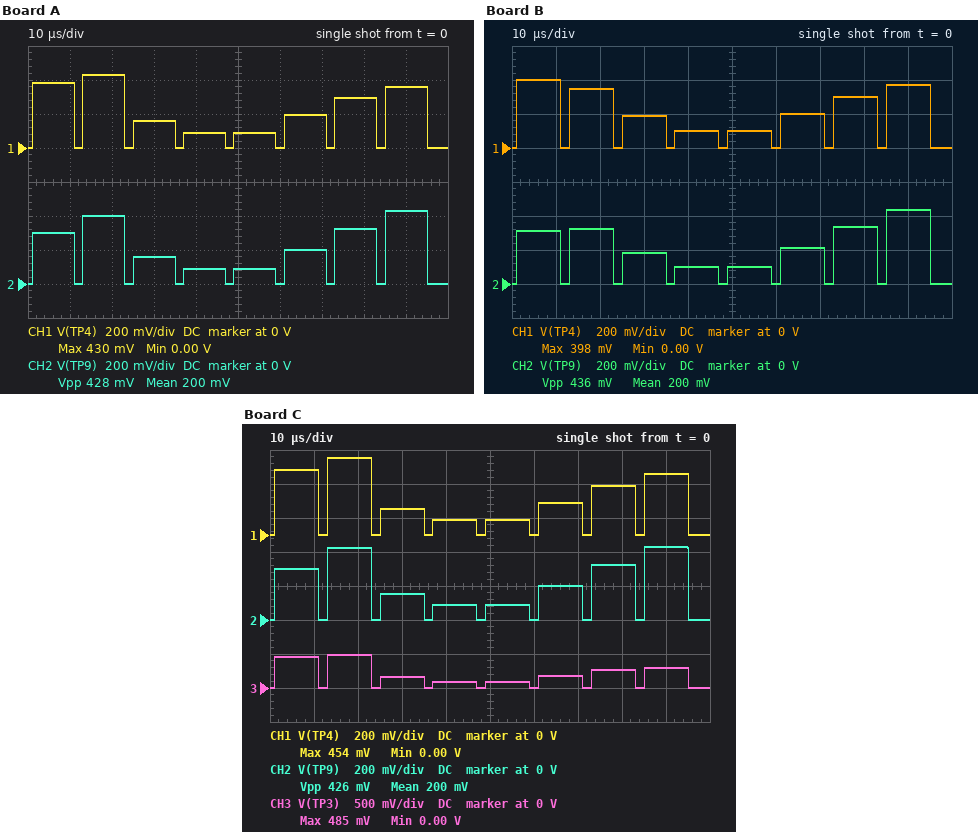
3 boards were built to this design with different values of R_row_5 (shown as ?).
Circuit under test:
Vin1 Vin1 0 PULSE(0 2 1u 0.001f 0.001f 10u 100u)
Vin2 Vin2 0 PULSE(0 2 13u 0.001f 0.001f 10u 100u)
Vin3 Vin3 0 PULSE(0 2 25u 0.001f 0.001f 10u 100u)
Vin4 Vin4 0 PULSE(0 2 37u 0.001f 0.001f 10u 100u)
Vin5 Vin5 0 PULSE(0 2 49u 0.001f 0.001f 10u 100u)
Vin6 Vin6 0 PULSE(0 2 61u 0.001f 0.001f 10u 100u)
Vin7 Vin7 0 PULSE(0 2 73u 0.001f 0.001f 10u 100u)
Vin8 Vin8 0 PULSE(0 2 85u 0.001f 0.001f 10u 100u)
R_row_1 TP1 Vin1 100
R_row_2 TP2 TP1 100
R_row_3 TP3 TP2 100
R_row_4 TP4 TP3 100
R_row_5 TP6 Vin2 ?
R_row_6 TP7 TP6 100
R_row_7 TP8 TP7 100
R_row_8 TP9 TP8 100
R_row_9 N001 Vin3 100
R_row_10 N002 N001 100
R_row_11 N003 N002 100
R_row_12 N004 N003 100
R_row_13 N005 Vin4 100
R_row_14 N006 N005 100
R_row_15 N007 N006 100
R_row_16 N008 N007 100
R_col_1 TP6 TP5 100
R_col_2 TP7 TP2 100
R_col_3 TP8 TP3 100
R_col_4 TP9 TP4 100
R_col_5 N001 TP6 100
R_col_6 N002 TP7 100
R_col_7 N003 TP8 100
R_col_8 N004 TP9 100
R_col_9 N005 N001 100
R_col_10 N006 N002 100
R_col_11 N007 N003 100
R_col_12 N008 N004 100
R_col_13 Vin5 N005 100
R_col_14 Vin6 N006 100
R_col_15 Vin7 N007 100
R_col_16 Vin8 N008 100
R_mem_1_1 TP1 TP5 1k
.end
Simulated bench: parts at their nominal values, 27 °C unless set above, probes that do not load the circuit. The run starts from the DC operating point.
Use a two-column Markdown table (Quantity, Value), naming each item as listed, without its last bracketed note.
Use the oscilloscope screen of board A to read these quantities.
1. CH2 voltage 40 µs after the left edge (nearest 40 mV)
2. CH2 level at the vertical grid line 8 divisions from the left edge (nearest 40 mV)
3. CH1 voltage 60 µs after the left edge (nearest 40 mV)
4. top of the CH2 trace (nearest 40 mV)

| Quantity | Value |
|---|---|
| CH2 voltage 40 µs after the left edge | 80 mV |
| CH2 level at the vertical grid line 8 divisions from the left edge | 320 mV |
| CH1 voltage 60 µs after the left edge | 0 V |
| top of the CH2 trace | 440 mV |
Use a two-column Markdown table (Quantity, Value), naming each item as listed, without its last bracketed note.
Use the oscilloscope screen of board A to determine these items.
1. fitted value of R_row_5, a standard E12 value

| Quantity | Value |
|---|---|
| fitted value of R_row_5, a standard E12 value | 39 Ω |
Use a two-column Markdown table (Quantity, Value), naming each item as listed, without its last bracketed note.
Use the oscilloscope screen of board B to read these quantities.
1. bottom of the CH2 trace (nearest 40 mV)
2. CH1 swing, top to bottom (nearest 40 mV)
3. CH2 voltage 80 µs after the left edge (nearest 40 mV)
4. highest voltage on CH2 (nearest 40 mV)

| Quantity | Value |
|---|---|
| bottom of the CH2 trace | 0 V |
| CH1 swing, top to bottom | 400 mV |
| CH2 voltage 80 µs after the left edge | 320 mV |
| highest voltage on CH2 | 440 mV |
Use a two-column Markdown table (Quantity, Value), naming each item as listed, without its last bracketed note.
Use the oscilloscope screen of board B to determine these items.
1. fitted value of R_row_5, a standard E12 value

| Quantity | Value |
|---|---|
| fitted value of R_row_5, a standard E12 value | 68 Ω |
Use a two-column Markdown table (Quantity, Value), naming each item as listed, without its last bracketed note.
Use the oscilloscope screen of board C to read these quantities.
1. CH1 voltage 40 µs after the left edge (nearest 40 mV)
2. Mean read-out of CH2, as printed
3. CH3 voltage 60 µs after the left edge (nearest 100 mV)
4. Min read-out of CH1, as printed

| Quantity | Value |
|---|---|
| CH1 voltage 40 µs after the left edge | 80 mV |
| Mean read-out of CH2, as printed | 200 mV |
| CH3 voltage 60 µs after the left edge | 0 V |
| Min read-out of CH1, as printed | 0.00 V |
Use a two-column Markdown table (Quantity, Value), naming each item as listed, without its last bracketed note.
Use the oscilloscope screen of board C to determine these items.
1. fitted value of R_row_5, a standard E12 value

| Quantity | Value |
|---|---|
| fitted value of R_row_5, a standard E12 value | 33 Ω |
